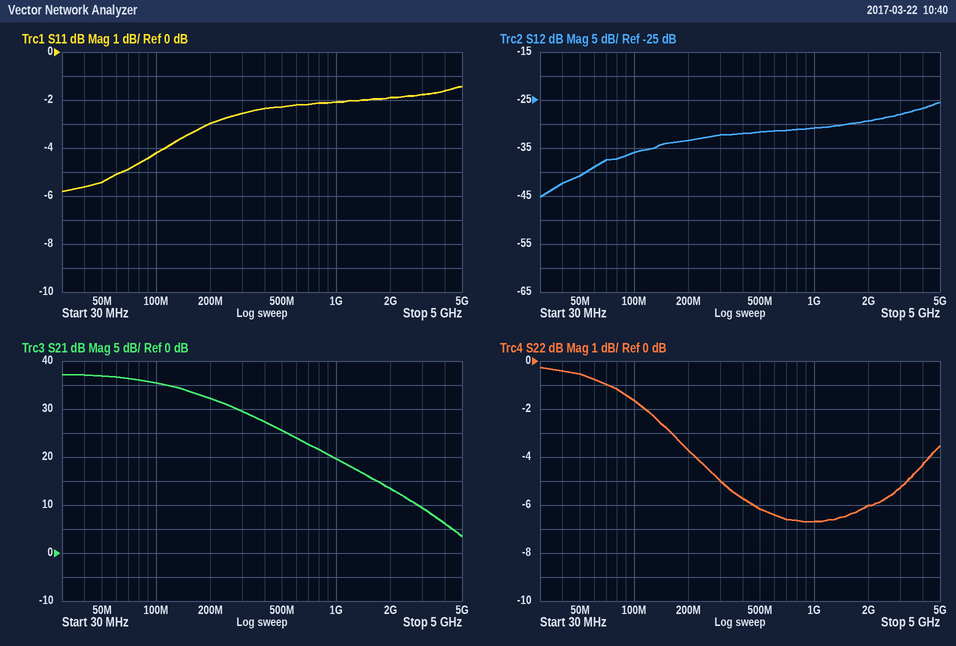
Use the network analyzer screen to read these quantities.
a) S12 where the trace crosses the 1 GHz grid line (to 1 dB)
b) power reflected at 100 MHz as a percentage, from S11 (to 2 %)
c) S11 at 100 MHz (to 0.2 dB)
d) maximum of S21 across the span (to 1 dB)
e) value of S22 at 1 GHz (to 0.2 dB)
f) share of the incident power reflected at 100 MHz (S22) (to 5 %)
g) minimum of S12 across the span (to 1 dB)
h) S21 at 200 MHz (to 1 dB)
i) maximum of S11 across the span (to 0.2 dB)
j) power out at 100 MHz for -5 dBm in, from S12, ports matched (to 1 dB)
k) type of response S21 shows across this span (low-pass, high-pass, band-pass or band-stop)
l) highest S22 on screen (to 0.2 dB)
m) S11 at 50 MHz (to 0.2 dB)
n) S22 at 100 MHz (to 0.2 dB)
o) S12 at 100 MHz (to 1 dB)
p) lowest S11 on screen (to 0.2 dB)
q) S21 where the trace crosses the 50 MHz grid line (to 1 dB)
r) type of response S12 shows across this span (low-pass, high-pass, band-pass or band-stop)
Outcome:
-31 dB
38 %
-4.2 dB
37 dB
-6.6 dB
70 %
-45 dB
32 dB
-1.4 dB
-41 dBm
low-pass
-0.2 dB
-5.4 dB
-1.6 dB
-36 dB
-5.8 dB
37 dB
high-pass
